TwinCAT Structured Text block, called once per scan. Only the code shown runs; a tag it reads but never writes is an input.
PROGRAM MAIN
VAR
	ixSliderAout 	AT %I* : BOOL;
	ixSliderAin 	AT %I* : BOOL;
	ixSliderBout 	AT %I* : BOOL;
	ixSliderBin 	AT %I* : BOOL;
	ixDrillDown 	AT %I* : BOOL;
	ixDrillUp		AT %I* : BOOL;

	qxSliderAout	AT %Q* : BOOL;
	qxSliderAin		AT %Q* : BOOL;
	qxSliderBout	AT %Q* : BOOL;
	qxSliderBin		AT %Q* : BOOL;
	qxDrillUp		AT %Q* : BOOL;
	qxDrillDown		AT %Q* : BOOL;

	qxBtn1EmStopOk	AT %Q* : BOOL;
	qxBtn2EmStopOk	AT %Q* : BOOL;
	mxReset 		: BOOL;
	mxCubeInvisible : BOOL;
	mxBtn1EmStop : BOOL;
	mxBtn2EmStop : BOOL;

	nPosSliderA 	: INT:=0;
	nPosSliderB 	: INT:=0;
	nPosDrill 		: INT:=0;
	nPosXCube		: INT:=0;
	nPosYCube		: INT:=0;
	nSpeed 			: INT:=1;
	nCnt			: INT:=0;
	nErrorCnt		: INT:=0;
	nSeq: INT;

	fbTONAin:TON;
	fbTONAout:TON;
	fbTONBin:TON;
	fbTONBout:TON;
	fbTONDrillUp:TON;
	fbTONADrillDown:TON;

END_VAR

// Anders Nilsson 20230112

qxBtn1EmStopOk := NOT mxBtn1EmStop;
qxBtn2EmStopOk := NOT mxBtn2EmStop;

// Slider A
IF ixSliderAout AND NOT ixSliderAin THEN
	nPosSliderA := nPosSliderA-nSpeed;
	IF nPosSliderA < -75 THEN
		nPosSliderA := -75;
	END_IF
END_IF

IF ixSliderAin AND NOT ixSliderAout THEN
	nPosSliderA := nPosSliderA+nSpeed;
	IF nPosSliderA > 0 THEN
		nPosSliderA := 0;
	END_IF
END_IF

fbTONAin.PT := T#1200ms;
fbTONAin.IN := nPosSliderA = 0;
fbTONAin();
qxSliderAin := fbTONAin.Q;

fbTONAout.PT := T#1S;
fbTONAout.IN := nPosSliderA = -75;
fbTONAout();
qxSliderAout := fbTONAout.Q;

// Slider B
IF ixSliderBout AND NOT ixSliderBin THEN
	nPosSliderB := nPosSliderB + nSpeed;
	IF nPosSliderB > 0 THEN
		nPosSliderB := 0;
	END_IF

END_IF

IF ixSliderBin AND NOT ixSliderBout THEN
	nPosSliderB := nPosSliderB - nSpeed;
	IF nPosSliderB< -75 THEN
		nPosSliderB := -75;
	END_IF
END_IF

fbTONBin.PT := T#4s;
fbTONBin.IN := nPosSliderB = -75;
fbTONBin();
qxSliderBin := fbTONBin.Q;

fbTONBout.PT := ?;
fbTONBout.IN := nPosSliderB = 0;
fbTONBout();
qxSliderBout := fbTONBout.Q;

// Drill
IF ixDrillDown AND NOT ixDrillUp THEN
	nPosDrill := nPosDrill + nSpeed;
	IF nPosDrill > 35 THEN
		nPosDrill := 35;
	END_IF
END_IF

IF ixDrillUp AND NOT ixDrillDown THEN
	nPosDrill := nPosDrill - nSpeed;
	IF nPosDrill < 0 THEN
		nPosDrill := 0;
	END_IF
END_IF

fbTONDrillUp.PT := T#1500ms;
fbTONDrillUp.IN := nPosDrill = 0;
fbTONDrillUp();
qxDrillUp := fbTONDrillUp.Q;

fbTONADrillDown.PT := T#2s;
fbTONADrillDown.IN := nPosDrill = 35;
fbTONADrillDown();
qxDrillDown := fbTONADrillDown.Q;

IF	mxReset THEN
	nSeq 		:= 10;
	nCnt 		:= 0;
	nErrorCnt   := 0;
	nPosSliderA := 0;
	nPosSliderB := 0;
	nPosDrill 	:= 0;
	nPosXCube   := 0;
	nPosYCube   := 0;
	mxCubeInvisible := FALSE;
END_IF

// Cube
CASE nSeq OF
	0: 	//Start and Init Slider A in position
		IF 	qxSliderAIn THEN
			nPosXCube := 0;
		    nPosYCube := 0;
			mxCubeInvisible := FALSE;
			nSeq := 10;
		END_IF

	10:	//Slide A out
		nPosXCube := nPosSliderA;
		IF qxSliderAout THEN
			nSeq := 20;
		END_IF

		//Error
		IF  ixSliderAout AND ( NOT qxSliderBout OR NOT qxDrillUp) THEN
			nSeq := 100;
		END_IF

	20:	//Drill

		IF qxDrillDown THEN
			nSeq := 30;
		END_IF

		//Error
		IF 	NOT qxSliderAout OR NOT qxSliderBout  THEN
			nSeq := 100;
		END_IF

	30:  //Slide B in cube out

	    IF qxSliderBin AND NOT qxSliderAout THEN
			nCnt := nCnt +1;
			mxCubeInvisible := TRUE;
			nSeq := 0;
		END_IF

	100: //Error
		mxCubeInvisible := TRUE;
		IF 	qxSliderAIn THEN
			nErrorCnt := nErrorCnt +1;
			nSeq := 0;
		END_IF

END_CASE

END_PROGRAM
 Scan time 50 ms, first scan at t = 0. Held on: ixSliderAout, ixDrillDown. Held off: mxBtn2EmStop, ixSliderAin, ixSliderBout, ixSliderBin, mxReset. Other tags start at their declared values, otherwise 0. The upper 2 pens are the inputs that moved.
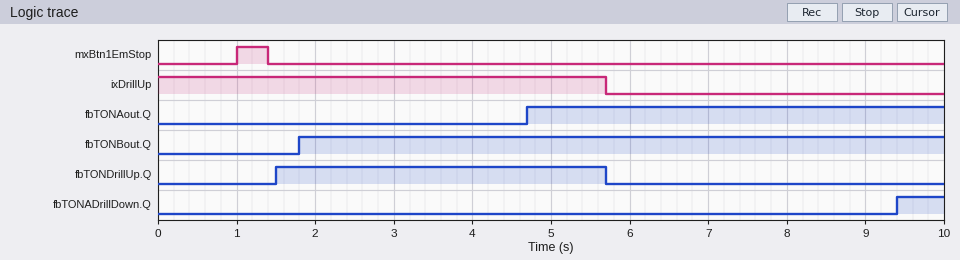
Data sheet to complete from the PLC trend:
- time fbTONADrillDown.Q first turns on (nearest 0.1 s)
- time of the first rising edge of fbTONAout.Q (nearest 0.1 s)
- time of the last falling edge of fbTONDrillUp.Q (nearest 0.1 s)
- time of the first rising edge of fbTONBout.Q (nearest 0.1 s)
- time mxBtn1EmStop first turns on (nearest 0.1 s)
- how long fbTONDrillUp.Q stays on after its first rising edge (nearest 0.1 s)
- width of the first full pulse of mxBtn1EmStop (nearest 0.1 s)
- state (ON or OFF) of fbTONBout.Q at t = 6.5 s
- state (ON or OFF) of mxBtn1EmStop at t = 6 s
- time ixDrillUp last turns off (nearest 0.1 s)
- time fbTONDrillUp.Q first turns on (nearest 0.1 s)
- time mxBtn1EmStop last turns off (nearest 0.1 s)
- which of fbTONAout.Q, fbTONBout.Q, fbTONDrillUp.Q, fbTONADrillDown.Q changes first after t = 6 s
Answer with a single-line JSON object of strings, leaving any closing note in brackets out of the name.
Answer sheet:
{"time fbTONADrillDown.Q first turns on": "9.4 s", "time of the first rising edge of fbTONAout.Q": "4.7 s", "time of the last falling edge of fbTONDrillUp.Q": "5.7 s", "time of the first rising edge of fbTONBout.Q": "1.8 s", "time mxBtn1EmStop first turns on": "1.0 s", "how long fbTONDrillUp.Q stays on after its first rising edge": "4.2 s", "width of the first full pulse of mxBtn1EmStop": "0.4 s", "state (ON or OFF) of fbTONBout.Q at t = 6.5 s": "ON", "state (ON or OFF) of mxBtn1EmStop at t = 6 s": "OFF", "time ixDrillUp last turns off": "5.7 s", "time fbTONDrillUp.Q first turns on": "1.5 s", "time mxBtn1EmStop last turns off": "1.4 s", "which of fbTONAout.Q, fbTONBout.Q, fbTONDrillUp.Q, fbTONADrillDown.Q changes first after t = 6 s": "fbTONADrillDown.Q"}
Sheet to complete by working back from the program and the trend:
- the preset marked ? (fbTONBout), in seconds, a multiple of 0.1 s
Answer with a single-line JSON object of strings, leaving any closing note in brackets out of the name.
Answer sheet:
{"the preset marked ? (fbTONBout), in seconds, a multiple of 0.1 s": "1.8 s"}
